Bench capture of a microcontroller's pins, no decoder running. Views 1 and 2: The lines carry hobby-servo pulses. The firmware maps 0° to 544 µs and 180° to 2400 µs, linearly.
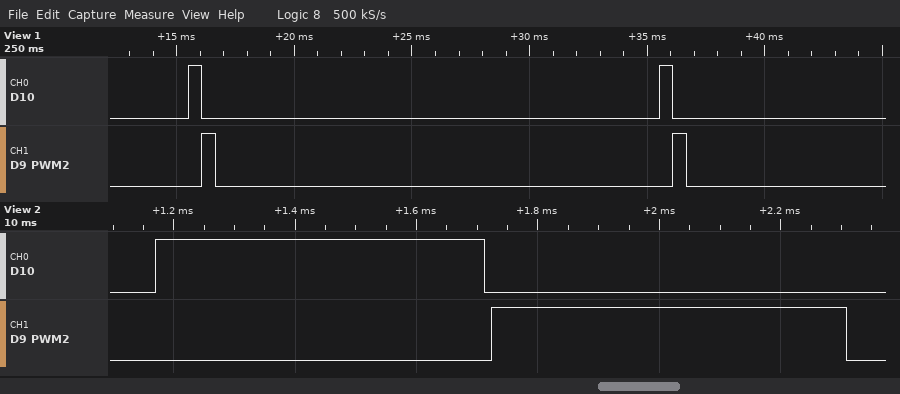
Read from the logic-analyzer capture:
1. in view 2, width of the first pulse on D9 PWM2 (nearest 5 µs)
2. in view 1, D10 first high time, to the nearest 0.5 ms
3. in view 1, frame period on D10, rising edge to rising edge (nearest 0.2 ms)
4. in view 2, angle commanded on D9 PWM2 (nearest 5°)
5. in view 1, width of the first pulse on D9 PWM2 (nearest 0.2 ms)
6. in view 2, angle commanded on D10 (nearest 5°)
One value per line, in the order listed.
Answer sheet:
585 µs
0.5 ms
20.0 ms
5°
0.6 ms
0°
